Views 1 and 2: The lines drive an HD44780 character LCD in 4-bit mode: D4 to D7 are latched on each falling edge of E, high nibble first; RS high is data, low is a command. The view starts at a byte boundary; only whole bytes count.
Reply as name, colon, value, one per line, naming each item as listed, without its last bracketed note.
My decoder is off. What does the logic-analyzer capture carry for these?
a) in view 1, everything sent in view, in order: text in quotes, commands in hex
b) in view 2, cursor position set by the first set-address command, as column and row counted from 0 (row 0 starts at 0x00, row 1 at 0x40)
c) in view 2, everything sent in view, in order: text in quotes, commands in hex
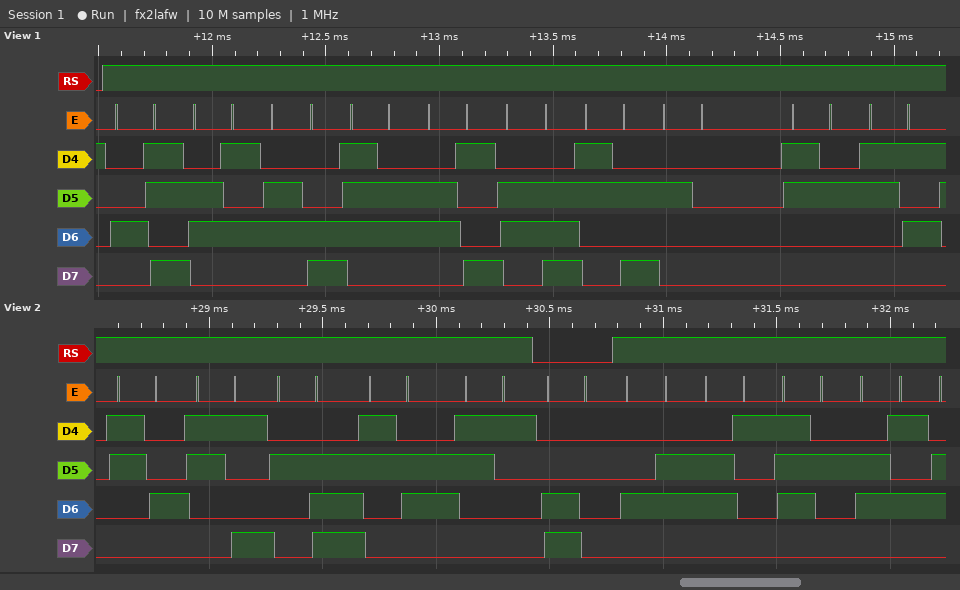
in view 1, everything sent in view, in order: text in quotes, commands in hex: "Kelvin: 25"
in view 2, cursor position set by the first set-address command, as column and row counted from 0: column 0, row 1
in view 2, everything sent in view, in order: text in quotes, commands in hex: "49.61" 0xC0 "Fare"
